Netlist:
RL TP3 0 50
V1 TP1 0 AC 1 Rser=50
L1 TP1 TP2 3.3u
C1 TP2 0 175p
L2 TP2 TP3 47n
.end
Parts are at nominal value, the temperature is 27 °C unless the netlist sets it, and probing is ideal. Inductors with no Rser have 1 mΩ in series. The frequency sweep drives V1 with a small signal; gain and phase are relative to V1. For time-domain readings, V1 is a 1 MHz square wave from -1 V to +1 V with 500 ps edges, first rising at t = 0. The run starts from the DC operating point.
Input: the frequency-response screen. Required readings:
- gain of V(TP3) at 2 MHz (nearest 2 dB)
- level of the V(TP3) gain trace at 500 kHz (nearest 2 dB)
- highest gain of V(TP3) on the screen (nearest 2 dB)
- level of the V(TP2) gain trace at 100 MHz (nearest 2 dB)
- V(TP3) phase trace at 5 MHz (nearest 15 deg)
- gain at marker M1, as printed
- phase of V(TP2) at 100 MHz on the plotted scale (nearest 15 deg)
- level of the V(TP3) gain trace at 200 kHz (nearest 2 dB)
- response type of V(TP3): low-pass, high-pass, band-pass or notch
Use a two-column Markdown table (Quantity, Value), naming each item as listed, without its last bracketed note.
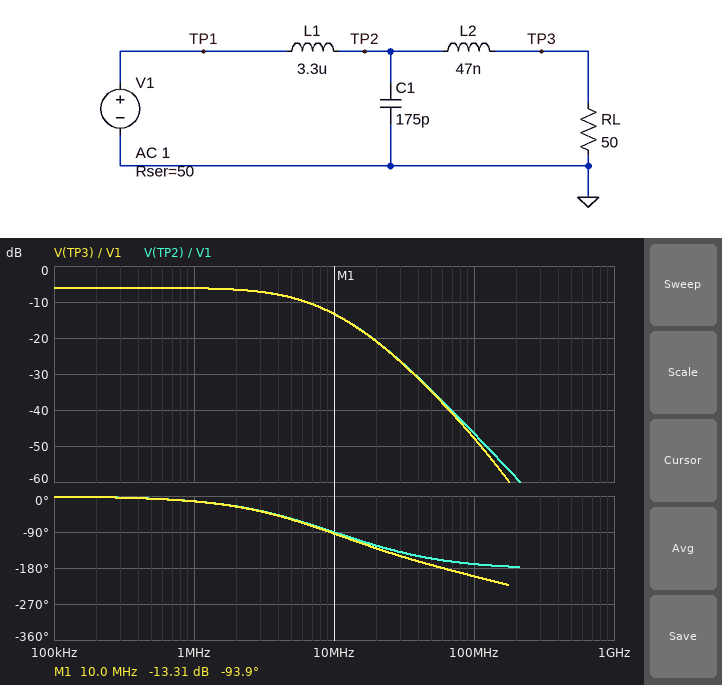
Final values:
| Quantity | Value |
|---|---|
| gain of V(TP3) at 2 MHz | -6 dB |
| level of the V(TP3) gain trace at 500 kHz | -6 dB |
| highest gain of V(TP3) on the screen | -6 dB |
| level of the V(TP2) gain trace at 100 MHz | -46 dB |
| V(TP3) phase trace at 5 MHz | -60 deg |
| gain at marker M1, as printed | -13.31 dB |
| phase of V(TP2) at 100 MHz on the plotted scale | -165 deg |
| level of the V(TP3) gain trace at 200 kHz | -6 dB |
| response type of V(TP3): low-pass, high-pass, band-pass or notch | low-pass |
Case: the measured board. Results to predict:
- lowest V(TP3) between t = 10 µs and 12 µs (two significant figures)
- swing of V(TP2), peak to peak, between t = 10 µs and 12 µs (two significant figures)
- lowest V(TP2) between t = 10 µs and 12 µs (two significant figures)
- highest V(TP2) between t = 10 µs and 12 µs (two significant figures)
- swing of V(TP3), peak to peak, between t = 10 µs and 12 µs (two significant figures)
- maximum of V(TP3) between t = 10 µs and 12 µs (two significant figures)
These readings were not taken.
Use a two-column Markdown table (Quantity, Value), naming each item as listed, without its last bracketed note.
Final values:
| Quantity | Value |
|---|---|
| lowest V(TP3) between t = 10 µs and 12 µs | -500 mV |
| swing of V(TP2), peak to peak, between t = 10 µs and 12 µs | 1.0 V |
| lowest V(TP2) between t = 10 µs and 12 µs | -500 mV |
| highest V(TP2) between t = 10 µs and 12 µs | 500 mV |
| swing of V(TP3), peak to peak, between t = 10 µs and 12 µs | 1.0 V |
| maximum of V(TP3) between t = 10 µs and 12 µs | 500 mV |
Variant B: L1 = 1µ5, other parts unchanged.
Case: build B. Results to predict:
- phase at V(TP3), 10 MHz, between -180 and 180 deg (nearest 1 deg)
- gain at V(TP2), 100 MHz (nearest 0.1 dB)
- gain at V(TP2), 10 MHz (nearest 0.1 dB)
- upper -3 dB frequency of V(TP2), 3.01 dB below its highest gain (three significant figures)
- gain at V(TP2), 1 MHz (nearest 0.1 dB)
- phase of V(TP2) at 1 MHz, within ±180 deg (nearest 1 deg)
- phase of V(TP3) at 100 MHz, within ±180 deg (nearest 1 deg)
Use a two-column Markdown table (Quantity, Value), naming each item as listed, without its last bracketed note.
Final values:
| Quantity | Value |
|---|---|
| phase at V(TP3), 10 MHz, between -180 and 180 deg | -69 deg |
| gain at V(TP2), 100 MHz | -39.6 dB |
| gain at V(TP2), 10 MHz | -8.3 dB |
| upper -3 dB frequency of V(TP2), 3.01 dB below its highest gain | 11.5 MHz |
| gain at V(TP2), 1 MHz | -6.0 dB |
| phase of V(TP2) at 1 MHz, within ±180 deg | -7 deg |
| phase of V(TP3) at 100 MHz, within ±180 deg | 161 deg |
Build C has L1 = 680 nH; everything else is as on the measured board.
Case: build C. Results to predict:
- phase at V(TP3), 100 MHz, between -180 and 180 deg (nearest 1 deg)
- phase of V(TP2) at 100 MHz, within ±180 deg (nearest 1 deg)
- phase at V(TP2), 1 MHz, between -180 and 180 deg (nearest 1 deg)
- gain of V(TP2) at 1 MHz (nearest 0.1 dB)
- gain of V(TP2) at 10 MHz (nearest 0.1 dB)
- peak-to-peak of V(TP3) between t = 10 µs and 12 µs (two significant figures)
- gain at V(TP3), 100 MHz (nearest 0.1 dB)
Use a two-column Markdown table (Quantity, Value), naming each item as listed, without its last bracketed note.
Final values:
| Quantity | Value |
|---|---|
| phase at V(TP3), 100 MHz, between -180 and 180 deg | 165 deg |
| phase of V(TP2) at 100 MHz, within ±180 deg | -165 deg |
| phase at V(TP2), 1 MHz, between -180 and 180 deg | -4 deg |
| gain of V(TP2) at 1 MHz | -6.0 dB |
| gain of V(TP2) at 10 MHz | -6.3 dB |
| peak-to-peak of V(TP3) between t = 10 µs and 12 µs | 1.1 V |
| gain at V(TP3), 100 MHz | -34.0 dB |
